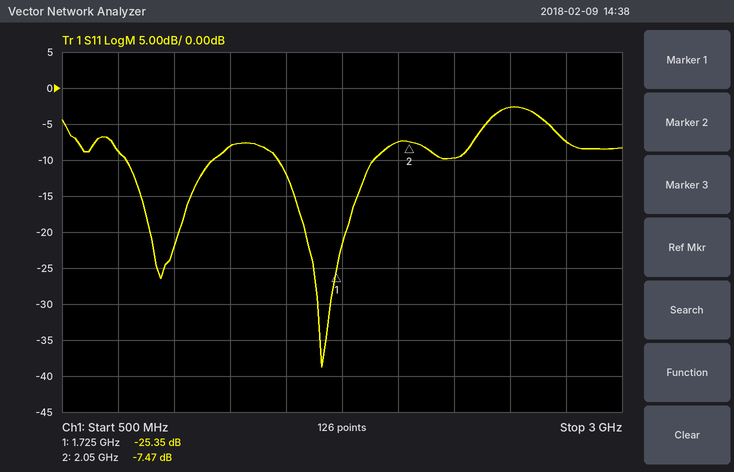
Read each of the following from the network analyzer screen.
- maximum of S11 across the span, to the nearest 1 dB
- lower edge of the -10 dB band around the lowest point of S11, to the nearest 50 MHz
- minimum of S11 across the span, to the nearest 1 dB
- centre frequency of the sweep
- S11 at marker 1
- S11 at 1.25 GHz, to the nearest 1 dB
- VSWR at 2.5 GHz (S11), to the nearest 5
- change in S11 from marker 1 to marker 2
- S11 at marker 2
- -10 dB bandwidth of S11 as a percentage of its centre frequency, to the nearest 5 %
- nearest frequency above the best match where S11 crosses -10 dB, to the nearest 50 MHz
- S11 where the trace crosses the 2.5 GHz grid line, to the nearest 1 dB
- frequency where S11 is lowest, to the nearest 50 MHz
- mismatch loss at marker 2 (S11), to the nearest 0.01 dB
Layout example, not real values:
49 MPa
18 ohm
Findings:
-3 dB
1.45 GHz
-39 dB
1.75 GHz
-25.35 dB
-8 dB
5
17.88 dB
-7.47 dB
25 %
1.90 GHz
-3 dB
1.65 GHz
0.86 dB
